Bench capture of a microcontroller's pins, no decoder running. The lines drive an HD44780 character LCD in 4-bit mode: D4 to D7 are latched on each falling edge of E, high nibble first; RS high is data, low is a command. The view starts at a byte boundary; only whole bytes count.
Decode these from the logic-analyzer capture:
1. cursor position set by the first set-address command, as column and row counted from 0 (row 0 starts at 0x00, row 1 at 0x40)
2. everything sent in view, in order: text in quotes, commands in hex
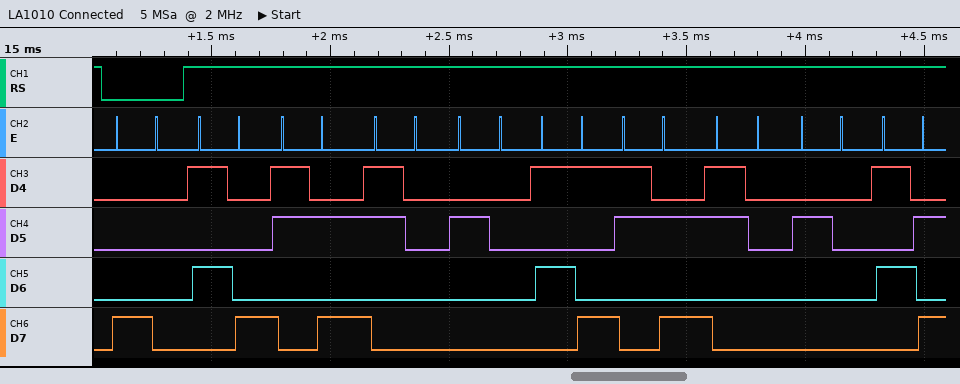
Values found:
column 0, row 0
0x80 "X:0 Y:0 Z"
